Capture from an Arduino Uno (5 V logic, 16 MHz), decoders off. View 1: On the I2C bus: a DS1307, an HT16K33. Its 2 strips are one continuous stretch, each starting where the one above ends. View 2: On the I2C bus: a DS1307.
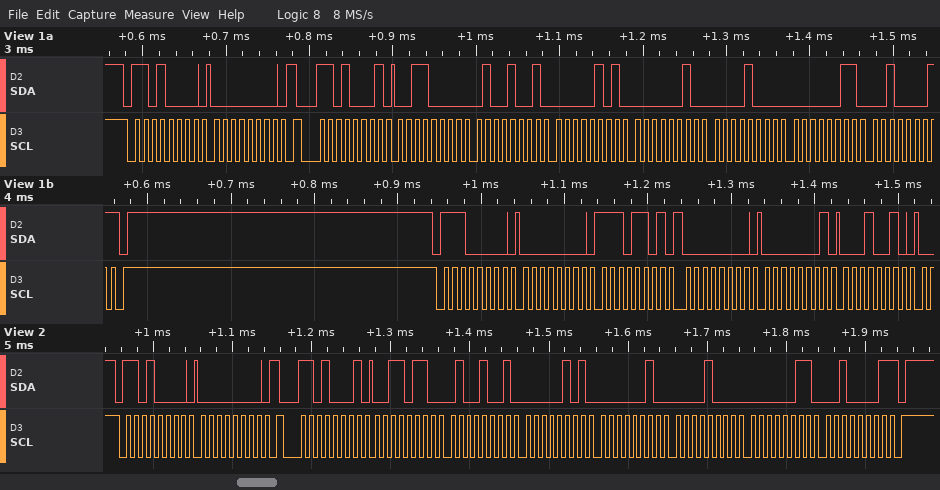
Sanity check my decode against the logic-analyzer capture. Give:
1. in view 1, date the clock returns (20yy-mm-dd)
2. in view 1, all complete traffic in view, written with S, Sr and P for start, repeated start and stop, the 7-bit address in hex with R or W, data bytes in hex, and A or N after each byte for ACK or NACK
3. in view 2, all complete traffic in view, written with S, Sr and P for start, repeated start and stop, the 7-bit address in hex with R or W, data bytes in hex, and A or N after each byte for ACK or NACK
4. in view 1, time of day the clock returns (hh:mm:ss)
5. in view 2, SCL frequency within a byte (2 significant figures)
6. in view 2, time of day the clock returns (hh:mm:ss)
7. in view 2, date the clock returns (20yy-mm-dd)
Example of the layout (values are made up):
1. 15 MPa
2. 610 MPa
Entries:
1. 2021-03-08
2. S 68W A 00 A Sr 68R A 30 A 49 A 05 A 02 A 08 A 03 A 21 N P S 70W A 00 A ED A 00 A 01 A 12 A
3. S 68W A 00 A Sr 68R A 36 A 49 A 05 A 02 A 08 A 03 A 21 N P
4. 05:49:30
5. 100 kHz
6. 05:49:36
7. 2021-03-08
